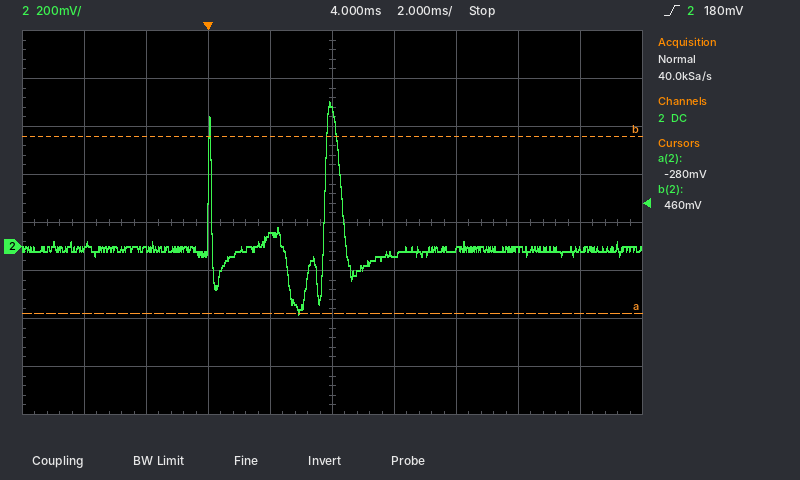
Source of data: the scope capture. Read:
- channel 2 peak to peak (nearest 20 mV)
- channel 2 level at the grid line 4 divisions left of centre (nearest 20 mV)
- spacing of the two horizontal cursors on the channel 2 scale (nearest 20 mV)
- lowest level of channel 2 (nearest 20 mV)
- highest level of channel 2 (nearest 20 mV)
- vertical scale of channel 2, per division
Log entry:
880 mV
0 mV
740 mV
-280 mV
600 mV
200 mV
